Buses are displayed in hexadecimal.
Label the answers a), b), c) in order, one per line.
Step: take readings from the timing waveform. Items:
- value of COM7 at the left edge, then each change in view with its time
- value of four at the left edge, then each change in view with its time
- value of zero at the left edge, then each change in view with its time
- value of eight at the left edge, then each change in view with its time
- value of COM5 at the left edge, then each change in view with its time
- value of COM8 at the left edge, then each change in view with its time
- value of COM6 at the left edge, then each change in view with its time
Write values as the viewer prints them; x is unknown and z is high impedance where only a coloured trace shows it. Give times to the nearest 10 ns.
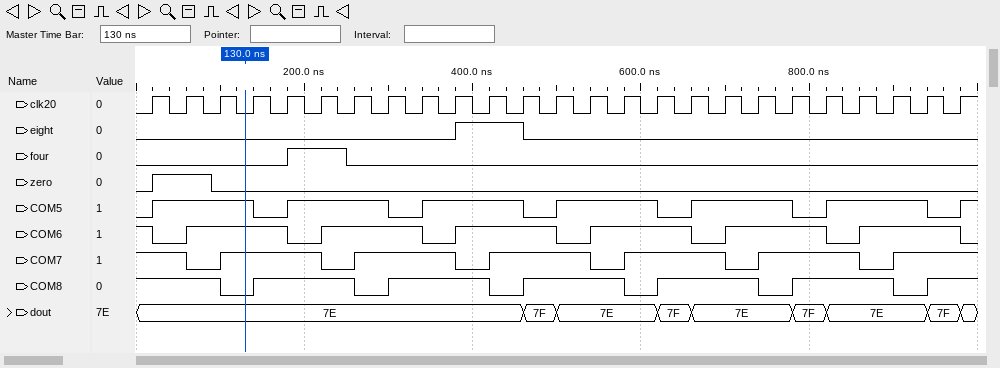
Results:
a) 1, 0 at 60 ns, 1 at 100 ns, 0 at 220 ns, 1 at 260 ns, 0 at 380 ns, 1 at 420 ns, 0 at 540 ns, 1 at 580 ns, 0 at 700 ns, 1 at 740 ns, 0 at 860 ns, 1 at 900 ns
b) 0, 1 at 180 ns, 0 at 250 ns
c) 0, 1 at 20 ns, 0 at 90 ns
d) 0, 1 at 380 ns, 0 at 460 ns
e) 0, 1 at 20 ns, 0 at 140 ns, 1 at 180 ns, 0 at 300 ns, 1 at 340 ns, 0 at 460 ns, 1 at 500 ns, 0 at 620 ns, 1 at 660 ns, 0 at 780 ns, 1 at 820 ns, 0 at 940 ns, 1 at 980 ns
f) 1, 0 at 100 ns, 1 at 140 ns, 0 at 260 ns, 1 at 300 ns, 0 at 420 ns, 1 at 460 ns, 0 at 580 ns, 1 at 620 ns, 0 at 740 ns, 1 at 780 ns, 0 at 900 ns, 1 at 940 ns
g) 1, 0 at 20 ns, 1 at 60 ns, 0 at 180 ns, 1 at 220 ns, 0 at 340 ns, 1 at 380 ns, 0 at 500 ns, 1 at 540 ns, 0 at 660 ns, 1 at 700 ns, 0 at 820 ns, 1 at 860 ns, 0 at 980 ns
